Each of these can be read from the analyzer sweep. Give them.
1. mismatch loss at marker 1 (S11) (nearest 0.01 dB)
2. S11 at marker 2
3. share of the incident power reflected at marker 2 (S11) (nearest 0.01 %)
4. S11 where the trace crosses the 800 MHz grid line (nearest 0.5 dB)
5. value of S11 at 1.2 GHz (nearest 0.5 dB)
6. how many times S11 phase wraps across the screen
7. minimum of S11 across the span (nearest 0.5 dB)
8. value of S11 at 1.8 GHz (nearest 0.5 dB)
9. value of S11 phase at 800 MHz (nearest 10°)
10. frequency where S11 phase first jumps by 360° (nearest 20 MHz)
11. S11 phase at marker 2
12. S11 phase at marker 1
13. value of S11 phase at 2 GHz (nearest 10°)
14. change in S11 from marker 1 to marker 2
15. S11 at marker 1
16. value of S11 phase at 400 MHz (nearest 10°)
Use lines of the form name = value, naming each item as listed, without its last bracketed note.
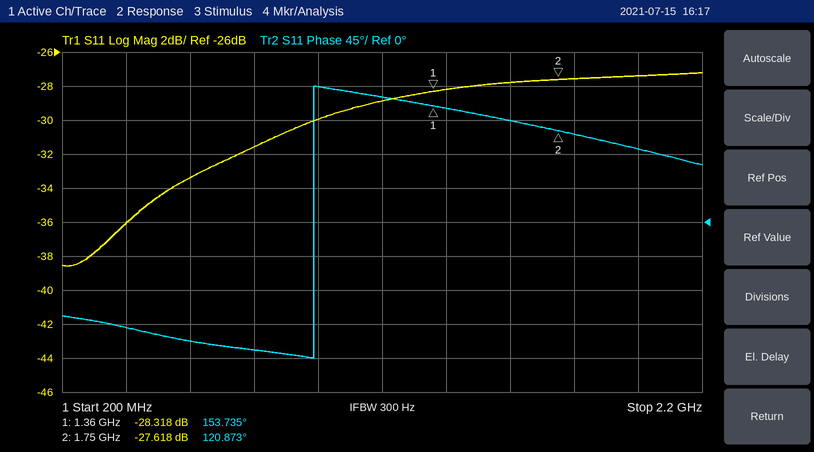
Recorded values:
mismatch loss at marker 1 (S11) = 0.01 dB
S11 at marker 2 = -27.618 dB
share of the incident power reflected at marker 2 (S11) = 0.17 %
S11 where the trace crosses the 800 MHz grid line = -31.5 dB
value of S11 at 1.2 GHz = -29.0 dB
how many times S11 phase wraps across the screen = 1
minimum of S11 across the span = -38.5 dB
value of S11 at 1.8 GHz = -27.5 dB
value of S11 phase at 800 MHz = -170°
frequency where S11 phase first jumps by 360° = 980 MHz
S11 phase at marker 2 = 120.873°
S11 phase at marker 1 = 153.735°
value of S11 phase at 2 GHz = 100°
change in S11 from marker 1 to marker 2 = 0.700 dB
S11 at marker 1 = -28.318 dB
value of S11 phase at 400 MHz = -140°
